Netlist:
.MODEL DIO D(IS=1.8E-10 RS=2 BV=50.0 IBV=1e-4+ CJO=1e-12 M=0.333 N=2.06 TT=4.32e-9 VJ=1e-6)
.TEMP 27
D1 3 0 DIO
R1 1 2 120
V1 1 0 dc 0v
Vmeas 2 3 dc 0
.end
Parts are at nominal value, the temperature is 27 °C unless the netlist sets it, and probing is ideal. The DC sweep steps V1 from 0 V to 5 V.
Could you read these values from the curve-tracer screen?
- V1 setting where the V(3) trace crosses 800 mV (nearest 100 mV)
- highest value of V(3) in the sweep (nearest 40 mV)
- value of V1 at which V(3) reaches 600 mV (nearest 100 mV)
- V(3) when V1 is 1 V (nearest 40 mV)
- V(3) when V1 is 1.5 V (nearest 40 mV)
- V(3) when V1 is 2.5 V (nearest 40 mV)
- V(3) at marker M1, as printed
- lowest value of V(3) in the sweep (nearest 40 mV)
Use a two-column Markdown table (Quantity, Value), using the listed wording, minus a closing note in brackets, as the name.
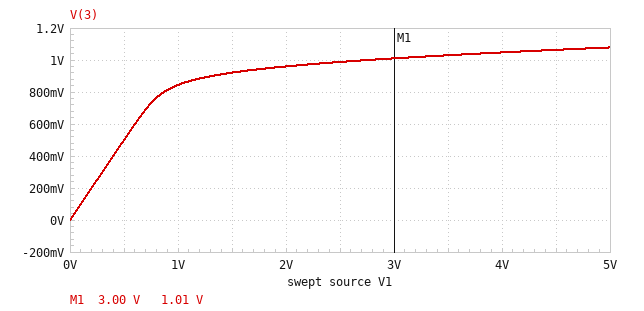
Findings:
| Quantity | Value |
|---|---|
| V1 setting where the V(3) trace crosses 800 mV | 900 mV |
| highest value of V(3) in the sweep | 1.08 V |
| value of V1 at which V(3) reaches 600 mV | 600 mV |
| V(3) when V1 is 1 V | 840 mV |
| V(3) when V1 is 1.5 V | 920 mV |
| V(3) when V1 is 2.5 V | 1.00 V |
| V(3) at marker M1, as printed | 1.01 V |
| lowest value of V(3) in the sweep | 0 V |
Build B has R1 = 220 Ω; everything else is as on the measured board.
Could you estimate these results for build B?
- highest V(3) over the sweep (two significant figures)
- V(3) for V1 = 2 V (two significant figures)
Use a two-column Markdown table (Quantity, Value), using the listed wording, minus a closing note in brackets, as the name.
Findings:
| Quantity | Value |
|---|---|
| highest V(3) over the sweep | 1.0 V |
| V(3) for V1 = 2 V | 920 mV |
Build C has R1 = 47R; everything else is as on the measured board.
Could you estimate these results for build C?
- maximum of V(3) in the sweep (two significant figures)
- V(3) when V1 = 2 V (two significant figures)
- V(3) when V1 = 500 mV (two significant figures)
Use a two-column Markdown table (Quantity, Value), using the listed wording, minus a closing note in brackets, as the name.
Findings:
| Quantity | Value |
|---|---|
| maximum of V(3) in the sweep | 1.2 V |
| V(3) when V1 = 2 V | 1.0 V |
| V(3) when V1 = 500 mV | 500 mV |
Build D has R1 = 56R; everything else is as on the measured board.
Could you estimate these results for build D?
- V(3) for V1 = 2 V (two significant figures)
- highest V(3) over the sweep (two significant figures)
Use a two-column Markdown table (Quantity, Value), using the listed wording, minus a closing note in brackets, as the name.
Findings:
| Quantity | Value |
|---|---|
| V(3) for V1 = 2 V | 1.0 V |
| highest V(3) over the sweep | 1.2 V |
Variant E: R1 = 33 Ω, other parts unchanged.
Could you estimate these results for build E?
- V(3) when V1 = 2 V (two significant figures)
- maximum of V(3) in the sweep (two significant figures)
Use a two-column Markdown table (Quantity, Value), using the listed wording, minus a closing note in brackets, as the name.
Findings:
| Quantity | Value |
|---|---|
| V(3) when V1 = 2 V | 1.1 V |
| maximum of V(3) in the sweep | 1.3 V |
